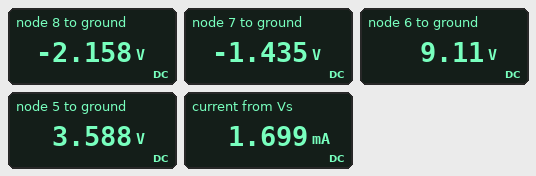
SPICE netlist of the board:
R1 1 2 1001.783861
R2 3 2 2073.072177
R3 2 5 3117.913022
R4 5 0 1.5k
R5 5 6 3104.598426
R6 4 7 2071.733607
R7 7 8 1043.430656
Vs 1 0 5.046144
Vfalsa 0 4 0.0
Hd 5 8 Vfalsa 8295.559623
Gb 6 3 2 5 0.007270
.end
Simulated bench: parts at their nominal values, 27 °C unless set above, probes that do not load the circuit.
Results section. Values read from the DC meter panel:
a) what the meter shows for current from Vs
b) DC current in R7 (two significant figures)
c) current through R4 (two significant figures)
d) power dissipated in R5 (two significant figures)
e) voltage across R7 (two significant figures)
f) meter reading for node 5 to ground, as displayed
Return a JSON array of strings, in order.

["1.699 mA", "690 µA", "2.4 mA", "9.8 mW", "720 mV", "3.588 V"]
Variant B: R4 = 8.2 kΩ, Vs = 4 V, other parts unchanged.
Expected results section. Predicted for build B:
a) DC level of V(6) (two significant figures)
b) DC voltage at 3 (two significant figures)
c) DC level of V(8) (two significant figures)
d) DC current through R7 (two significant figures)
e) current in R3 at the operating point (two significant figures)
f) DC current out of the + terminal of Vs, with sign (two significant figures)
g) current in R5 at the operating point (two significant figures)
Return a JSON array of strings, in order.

["3.3 V", "5.0 V", "-2.6 V", "820 µA", "14 µA", "-300 µA", "320 µA"]
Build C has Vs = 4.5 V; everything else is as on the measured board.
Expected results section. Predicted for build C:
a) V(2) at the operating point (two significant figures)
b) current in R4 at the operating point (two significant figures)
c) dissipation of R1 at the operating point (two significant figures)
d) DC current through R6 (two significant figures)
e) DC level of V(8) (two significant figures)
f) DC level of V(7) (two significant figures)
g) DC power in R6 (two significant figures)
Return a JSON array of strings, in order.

["3.0 V", "2.1 mA", "2.3 mW", "620 µA", "-1.9 V", "-1.3 V", "790 µW"]
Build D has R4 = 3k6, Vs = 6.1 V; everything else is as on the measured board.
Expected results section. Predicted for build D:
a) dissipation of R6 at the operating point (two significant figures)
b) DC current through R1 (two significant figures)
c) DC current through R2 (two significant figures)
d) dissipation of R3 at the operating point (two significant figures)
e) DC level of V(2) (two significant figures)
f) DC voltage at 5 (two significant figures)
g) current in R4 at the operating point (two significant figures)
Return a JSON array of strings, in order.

["2.5 mW", "480 µA", "500 µA", "1.5 µW", "5.6 V", "5.7 V", "1.6 mA"]
